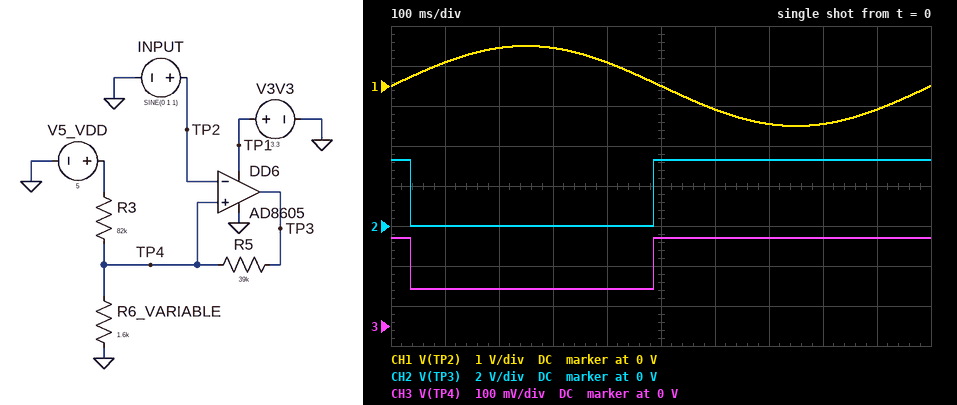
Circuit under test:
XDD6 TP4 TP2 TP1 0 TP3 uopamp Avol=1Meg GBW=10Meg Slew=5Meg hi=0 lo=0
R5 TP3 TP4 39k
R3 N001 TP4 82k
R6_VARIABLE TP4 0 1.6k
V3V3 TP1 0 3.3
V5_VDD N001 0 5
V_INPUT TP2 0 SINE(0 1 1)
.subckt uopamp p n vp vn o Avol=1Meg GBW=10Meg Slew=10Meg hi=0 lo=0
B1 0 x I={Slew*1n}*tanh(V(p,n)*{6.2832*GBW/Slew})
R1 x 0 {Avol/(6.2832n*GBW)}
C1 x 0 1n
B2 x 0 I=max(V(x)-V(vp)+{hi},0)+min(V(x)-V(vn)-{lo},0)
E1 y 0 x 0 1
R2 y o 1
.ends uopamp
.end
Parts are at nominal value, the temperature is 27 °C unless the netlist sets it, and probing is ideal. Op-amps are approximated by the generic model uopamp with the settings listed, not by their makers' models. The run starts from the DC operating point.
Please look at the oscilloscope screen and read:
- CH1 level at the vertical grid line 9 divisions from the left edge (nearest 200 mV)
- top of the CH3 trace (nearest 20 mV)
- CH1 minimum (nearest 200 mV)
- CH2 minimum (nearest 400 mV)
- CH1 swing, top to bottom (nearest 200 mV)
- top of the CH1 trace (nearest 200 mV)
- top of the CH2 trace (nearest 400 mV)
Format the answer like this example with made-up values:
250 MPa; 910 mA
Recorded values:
-600 mV; 220 mV; -1.0 V; 0 V; 2.0 V; 1.0 V; 3.2 V
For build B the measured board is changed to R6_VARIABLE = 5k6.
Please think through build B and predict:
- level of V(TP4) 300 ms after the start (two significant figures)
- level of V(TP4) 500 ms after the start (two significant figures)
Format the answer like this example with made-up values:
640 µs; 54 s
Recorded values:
280 mV; 670 mV
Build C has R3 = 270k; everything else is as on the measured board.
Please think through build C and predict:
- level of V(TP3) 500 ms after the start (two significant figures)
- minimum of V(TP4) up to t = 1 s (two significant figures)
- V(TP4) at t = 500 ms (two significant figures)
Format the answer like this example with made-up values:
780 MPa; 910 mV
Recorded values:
3.3 V; 28 mV; 160 mV
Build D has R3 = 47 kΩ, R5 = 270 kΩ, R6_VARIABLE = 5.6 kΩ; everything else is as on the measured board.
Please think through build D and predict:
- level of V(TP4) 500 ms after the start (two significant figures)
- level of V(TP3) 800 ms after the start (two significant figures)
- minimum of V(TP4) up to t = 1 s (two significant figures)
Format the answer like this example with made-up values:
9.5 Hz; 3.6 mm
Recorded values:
580 mV; 3.3 V; 520 mV
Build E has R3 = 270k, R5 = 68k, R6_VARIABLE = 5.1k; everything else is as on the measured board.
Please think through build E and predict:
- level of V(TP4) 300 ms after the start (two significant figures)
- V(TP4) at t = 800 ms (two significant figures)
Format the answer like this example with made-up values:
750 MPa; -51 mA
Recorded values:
86 mV; 310 mV
